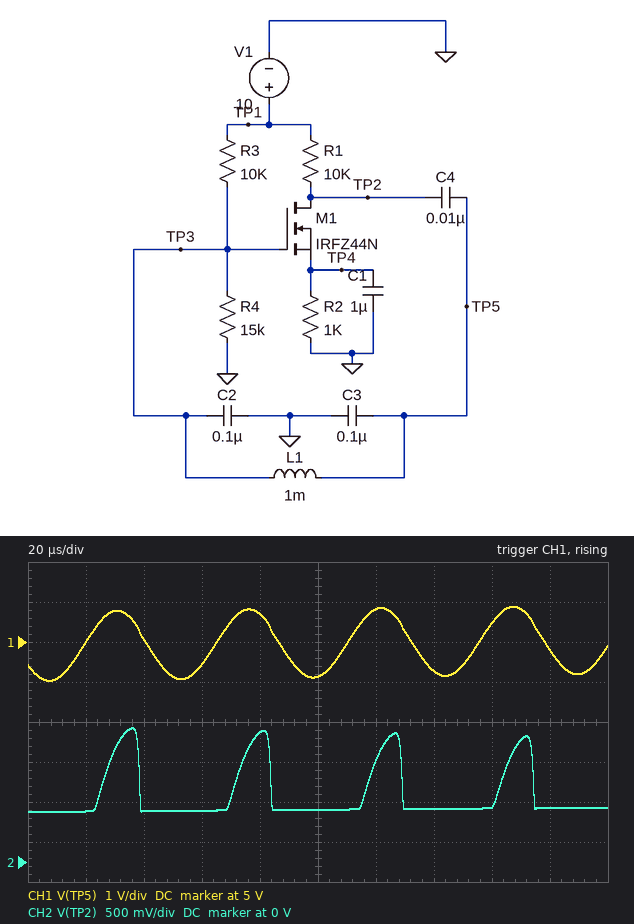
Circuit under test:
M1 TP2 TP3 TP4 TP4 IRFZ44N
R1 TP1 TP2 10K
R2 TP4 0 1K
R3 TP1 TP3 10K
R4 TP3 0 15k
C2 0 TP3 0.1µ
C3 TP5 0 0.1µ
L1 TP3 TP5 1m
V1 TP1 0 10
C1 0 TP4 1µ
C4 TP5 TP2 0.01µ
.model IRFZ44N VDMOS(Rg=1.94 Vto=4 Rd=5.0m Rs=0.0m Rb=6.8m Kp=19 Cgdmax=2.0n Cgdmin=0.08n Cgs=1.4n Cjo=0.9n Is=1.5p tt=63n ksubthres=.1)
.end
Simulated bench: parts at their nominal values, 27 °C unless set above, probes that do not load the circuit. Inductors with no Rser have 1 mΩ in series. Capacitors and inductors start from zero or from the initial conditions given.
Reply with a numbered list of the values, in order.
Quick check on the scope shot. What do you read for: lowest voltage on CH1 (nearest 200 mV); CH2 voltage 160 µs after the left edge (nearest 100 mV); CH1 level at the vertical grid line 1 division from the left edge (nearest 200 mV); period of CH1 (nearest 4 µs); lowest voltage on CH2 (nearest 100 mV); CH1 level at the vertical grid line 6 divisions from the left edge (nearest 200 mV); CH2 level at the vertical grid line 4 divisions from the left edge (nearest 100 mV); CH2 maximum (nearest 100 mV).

1. 4.0 V
2. 700 mV
3. 5.0 V
4. 44 µs
5. 600 mV
6. 5.8 V
7. 1.6 V
8. 1.7 V
